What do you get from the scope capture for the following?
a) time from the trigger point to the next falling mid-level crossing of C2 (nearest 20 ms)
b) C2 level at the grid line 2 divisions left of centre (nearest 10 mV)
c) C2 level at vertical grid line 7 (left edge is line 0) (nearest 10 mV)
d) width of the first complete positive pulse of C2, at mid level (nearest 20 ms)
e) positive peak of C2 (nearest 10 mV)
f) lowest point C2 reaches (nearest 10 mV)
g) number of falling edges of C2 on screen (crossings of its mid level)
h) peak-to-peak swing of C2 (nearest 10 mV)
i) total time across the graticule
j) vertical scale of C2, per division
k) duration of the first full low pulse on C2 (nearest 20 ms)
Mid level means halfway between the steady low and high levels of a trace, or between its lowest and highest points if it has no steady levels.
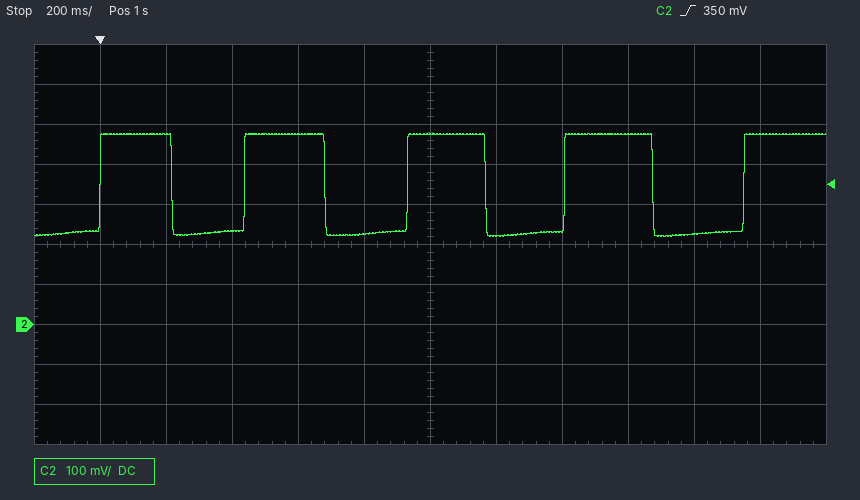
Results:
220 ms
480 mV
220 mV
220 ms
480 mV
220 mV
4
260 mV
2.4 s
100 mV
220 ms
